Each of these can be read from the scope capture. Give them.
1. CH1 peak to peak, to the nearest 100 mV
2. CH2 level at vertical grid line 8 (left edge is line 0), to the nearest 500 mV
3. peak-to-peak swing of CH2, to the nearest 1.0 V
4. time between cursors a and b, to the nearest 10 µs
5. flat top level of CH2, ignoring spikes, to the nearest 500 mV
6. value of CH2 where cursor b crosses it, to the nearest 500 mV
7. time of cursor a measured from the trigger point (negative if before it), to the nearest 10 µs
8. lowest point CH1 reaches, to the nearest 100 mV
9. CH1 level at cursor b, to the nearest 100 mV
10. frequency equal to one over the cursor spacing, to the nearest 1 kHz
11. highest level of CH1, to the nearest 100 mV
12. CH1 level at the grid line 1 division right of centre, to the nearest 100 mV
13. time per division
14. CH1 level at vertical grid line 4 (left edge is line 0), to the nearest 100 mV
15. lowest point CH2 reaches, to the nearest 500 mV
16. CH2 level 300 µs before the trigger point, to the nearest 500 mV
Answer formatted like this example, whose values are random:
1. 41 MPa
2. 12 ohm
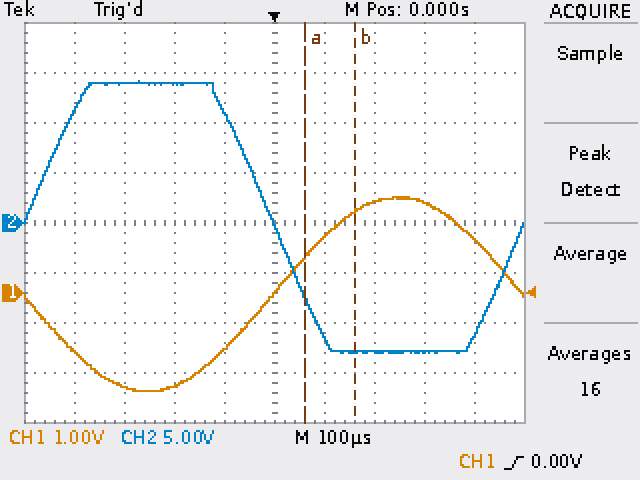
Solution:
1. 3.9 V
2. -13.0 V
3. 27.0 V
4. 100 µs
5. 14.0 V
6. -13.0 V
7. +60 µs
8. -2.0 V
9. 1.6 V
10. 10 kHz
11. 1.9 V
12. 1.1 V
13. 100 µs
14. -1.1 V
15. -13.0 V
16. 14.0 V
